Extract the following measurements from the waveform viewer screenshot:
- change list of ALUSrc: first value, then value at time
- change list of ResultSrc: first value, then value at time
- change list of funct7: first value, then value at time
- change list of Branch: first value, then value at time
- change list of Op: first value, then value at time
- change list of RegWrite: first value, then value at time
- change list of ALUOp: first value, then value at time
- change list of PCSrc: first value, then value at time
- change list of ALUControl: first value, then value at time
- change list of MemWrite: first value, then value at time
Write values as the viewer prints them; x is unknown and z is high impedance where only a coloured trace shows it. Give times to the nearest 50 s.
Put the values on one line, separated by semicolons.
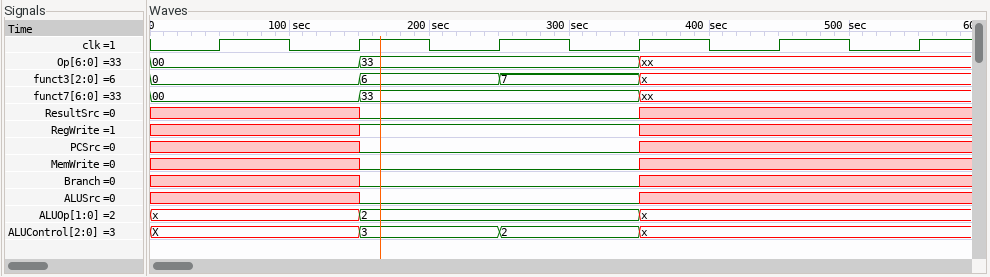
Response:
x, 0 at 150 s, x at 350 s; x, 0 at 150 s, x at 350 s; 00, 33 at 150 s, xx at 350 s; x, 0 at 150 s, x at 350 s; 00, 33 at 150 s, xx at 350 s; x, 1 at 150 s, x at 350 s; x, 2 at 150 s, x at 350 s; x, 0 at 150 s, x at 350 s; X, 3 at 150 s, 2 at 250 s, x at 350 s; x, 0 at 150 s, x at 350 s
